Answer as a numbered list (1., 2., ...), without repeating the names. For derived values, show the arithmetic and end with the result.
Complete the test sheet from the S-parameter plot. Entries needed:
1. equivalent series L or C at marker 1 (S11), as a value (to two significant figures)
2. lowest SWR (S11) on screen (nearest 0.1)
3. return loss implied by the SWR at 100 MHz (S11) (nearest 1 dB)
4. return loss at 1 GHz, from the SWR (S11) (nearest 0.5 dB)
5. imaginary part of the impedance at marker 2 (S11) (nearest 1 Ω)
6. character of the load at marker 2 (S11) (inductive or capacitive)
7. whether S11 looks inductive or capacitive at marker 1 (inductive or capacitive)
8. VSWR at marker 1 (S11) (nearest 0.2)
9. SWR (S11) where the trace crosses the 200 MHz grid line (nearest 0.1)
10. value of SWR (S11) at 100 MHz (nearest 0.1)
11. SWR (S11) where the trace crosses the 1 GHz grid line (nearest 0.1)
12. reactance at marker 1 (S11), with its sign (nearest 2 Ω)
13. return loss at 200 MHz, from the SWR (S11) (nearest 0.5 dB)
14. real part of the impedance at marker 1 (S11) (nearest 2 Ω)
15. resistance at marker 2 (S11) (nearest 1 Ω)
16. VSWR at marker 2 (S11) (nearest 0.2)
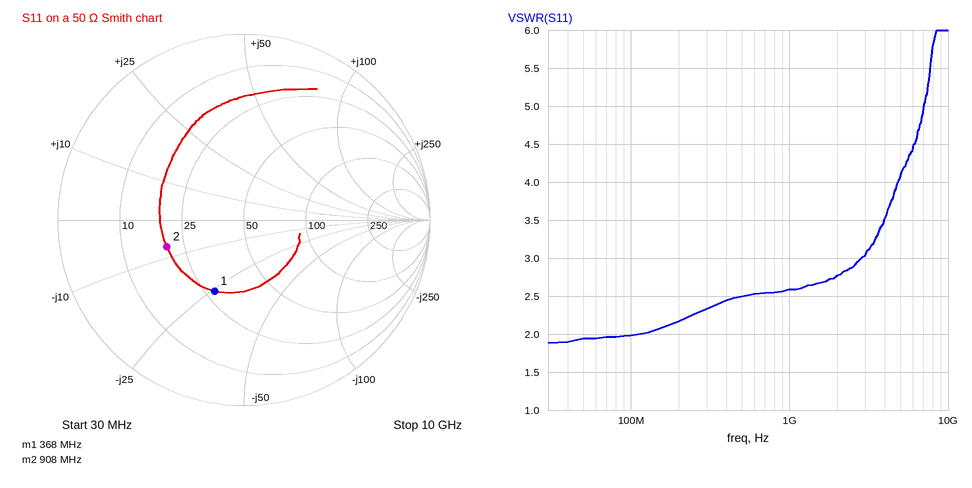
1. C = 1/(2π × 368 MHz × 26 Ω) ≈ 17 pF
2. 1.9
3. −20 log10((2 − 1)/(2 + 1)) ≈ 10 dB
4. −20 log10((2.6 − 1)/(2.6 + 1)) ≈ 7.0 dB
5. -7 Ω
6. capacitive
7. capacitive
8. 2.4
9. 2.2
10. 2.0
11. 2.6
12. -26 Ω
13. −20 log10((2.2 − 1)/(2.2 + 1)) ≈ 8.5 dB
14. 28 Ω
15. 20 Ω
16. 2.6
